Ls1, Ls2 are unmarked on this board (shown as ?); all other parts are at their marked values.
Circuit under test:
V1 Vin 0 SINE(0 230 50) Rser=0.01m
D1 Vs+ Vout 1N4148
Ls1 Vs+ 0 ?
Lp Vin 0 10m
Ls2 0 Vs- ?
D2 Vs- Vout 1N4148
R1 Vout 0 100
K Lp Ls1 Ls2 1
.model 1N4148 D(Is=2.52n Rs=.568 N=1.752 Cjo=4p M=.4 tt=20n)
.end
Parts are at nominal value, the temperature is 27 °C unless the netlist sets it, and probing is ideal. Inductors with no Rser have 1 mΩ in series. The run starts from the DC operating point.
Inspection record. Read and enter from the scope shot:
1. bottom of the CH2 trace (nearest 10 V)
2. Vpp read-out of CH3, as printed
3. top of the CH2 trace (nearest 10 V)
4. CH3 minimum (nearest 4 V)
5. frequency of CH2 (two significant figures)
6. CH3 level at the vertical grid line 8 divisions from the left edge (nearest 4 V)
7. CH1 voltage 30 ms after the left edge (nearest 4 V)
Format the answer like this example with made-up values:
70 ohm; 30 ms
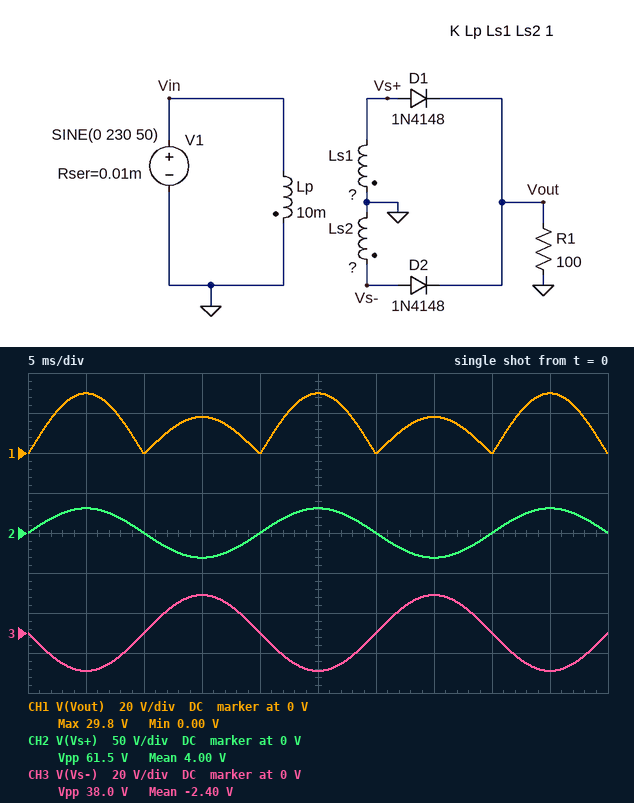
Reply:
-30 V; 38.0 V; 30 V; -20 V; 50 Hz; 0 V; 0 V
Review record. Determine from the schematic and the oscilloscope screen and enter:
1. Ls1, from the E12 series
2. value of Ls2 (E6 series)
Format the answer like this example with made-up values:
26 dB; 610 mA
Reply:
180 µH; 68 µH
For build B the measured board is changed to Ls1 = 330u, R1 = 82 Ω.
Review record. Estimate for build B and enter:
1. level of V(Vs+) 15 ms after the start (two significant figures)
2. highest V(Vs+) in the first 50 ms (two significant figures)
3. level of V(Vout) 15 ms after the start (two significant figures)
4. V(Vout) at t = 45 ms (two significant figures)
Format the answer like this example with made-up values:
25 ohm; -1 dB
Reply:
-42 V; 42 V; 18 V; 41 V
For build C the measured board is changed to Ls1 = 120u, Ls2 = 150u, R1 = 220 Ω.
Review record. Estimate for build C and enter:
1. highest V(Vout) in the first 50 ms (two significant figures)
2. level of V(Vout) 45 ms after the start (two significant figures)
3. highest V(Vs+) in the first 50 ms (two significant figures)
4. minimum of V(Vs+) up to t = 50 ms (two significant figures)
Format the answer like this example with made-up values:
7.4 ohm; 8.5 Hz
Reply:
27 V; 24 V; 25 V; -25 V
